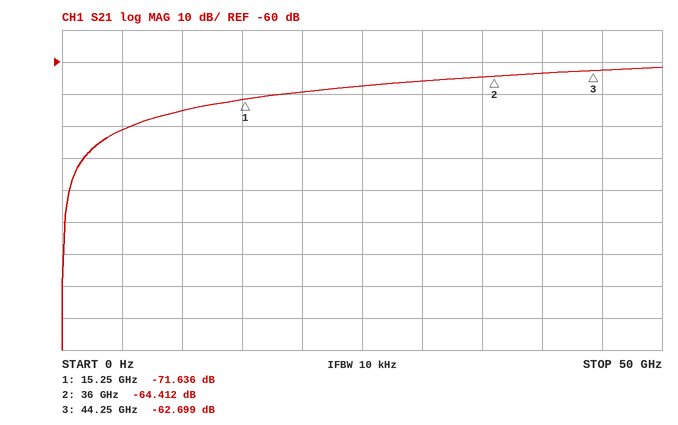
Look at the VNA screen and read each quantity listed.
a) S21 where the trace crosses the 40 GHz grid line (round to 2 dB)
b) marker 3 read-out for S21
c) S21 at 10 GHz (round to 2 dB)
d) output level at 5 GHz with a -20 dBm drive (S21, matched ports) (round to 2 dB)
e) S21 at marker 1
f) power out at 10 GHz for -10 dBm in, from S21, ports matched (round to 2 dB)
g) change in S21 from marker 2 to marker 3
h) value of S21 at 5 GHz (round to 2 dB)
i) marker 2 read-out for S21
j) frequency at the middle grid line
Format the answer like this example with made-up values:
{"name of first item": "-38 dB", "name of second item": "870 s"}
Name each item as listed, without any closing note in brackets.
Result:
{"S21 where the trace crosses the 40 GHz grid line": "-64 dB", "marker 3 read-out for S21": "-62.699 dB", "S21 at 10 GHz": "-76 dB", "output level at 5 GHz with a -20 dBm drive (S21, matched ports)": "-102 dBm", "S21 at marker 1": "-71.636 dB", "power out at 10 GHz for -10 dBm in, from S21, ports matched": "-86 dBm", "change in S21 from marker 2 to marker 3": "1.713 dB", "value of S21 at 5 GHz": "-82 dB", "marker 2 read-out for S21": "-64.412 dB", "frequency at the middle grid line": "25 GHz"}
